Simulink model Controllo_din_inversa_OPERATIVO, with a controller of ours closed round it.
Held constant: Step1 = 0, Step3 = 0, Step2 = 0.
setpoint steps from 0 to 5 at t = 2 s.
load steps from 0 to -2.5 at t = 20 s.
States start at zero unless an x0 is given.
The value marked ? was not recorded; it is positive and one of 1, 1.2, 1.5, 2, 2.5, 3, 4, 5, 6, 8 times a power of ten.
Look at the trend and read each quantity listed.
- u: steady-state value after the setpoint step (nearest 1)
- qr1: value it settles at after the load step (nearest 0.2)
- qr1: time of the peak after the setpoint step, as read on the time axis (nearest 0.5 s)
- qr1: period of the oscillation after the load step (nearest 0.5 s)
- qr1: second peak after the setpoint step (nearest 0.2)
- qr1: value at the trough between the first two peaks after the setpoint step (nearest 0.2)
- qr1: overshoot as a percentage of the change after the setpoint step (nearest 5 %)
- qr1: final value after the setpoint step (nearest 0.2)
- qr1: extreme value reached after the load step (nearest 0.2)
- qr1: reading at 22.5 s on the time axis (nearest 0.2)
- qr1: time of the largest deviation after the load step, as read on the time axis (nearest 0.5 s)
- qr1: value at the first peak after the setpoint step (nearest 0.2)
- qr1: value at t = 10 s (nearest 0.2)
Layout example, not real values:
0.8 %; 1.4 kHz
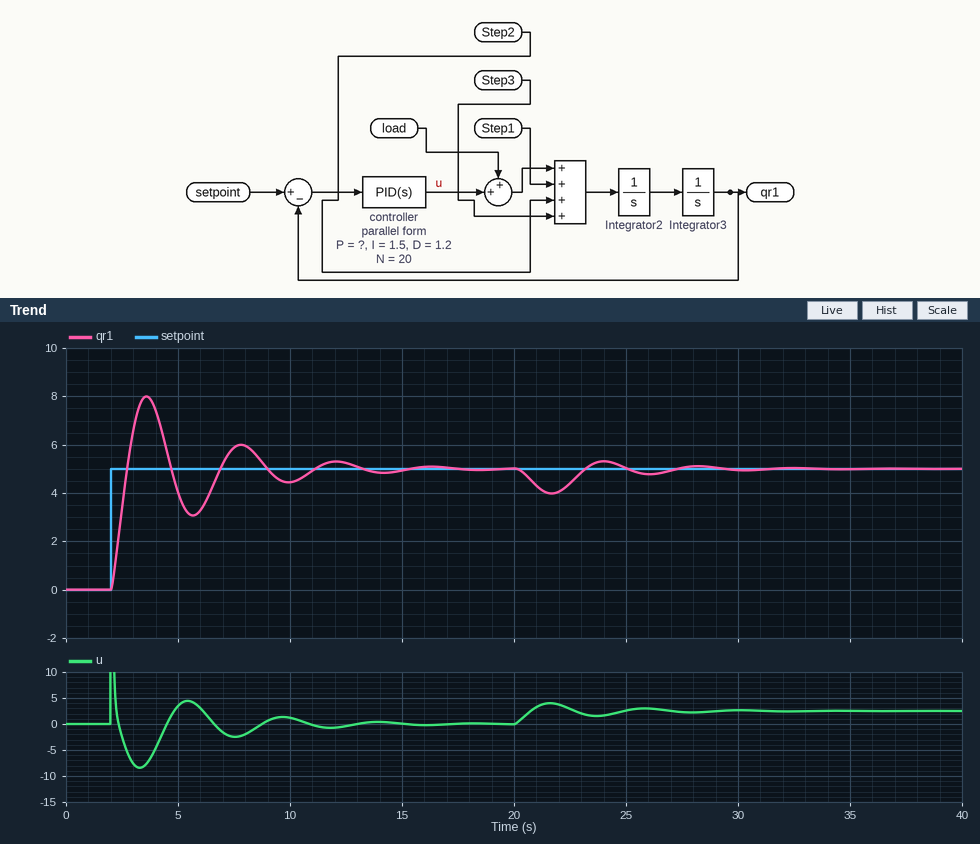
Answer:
0; 5.0; 3.5 s; 4.5 s; 6.0; 3.0; 60 %; 5.0; 4.0; 4.4; 21.5 s; 8.0; 4.4
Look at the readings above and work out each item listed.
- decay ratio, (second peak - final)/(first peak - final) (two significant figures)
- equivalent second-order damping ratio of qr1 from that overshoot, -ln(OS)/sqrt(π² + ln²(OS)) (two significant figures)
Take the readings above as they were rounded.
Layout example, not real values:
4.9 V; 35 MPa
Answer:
0.33; 0.16
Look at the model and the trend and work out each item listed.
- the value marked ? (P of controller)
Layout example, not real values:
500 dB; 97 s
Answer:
2.5
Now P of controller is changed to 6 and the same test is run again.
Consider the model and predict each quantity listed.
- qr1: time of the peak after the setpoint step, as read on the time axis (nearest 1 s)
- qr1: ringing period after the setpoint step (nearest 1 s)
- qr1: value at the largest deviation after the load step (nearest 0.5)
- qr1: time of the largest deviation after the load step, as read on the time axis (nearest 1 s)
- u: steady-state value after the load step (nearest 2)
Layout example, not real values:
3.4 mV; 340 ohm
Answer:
3 s; 3 s; 4.5; 21 s; 2
